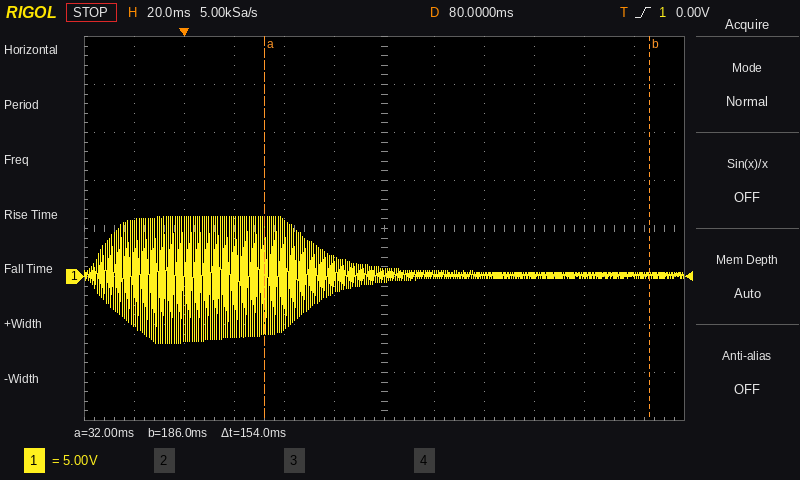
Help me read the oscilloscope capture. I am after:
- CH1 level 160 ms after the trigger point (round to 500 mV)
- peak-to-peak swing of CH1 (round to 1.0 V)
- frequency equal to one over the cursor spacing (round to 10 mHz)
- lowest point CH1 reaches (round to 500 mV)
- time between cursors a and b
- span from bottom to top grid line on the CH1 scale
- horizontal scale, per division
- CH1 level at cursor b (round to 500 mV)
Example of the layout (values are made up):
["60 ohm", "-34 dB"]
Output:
["0.0 V", "13.0 V", "6.49 Hz", "-7.0 V", "154 ms", "40 V", "20 ms", "0.0 V"]
